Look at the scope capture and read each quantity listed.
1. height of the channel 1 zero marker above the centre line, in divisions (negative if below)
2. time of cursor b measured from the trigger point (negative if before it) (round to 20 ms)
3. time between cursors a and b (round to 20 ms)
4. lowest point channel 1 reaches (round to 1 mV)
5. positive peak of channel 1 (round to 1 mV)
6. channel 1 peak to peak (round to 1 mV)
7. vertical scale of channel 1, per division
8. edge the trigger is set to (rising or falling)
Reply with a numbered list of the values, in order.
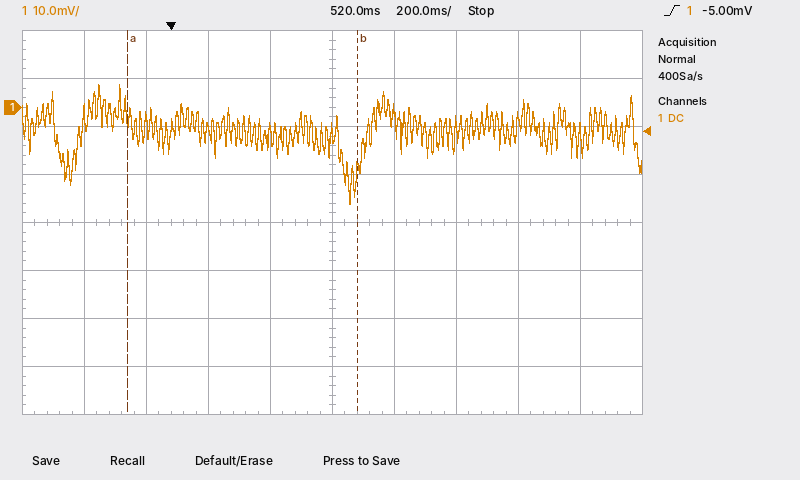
1. +2.4 div
2. +600 ms
3. 740 ms
4. -20 mV
5. 5 mV
6. 25 mV
7. 10 mV
8. rising
